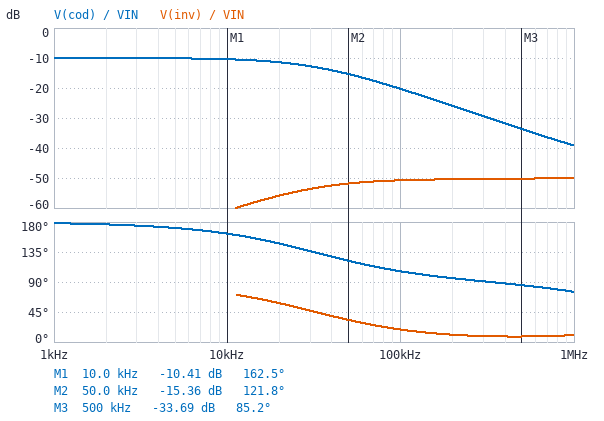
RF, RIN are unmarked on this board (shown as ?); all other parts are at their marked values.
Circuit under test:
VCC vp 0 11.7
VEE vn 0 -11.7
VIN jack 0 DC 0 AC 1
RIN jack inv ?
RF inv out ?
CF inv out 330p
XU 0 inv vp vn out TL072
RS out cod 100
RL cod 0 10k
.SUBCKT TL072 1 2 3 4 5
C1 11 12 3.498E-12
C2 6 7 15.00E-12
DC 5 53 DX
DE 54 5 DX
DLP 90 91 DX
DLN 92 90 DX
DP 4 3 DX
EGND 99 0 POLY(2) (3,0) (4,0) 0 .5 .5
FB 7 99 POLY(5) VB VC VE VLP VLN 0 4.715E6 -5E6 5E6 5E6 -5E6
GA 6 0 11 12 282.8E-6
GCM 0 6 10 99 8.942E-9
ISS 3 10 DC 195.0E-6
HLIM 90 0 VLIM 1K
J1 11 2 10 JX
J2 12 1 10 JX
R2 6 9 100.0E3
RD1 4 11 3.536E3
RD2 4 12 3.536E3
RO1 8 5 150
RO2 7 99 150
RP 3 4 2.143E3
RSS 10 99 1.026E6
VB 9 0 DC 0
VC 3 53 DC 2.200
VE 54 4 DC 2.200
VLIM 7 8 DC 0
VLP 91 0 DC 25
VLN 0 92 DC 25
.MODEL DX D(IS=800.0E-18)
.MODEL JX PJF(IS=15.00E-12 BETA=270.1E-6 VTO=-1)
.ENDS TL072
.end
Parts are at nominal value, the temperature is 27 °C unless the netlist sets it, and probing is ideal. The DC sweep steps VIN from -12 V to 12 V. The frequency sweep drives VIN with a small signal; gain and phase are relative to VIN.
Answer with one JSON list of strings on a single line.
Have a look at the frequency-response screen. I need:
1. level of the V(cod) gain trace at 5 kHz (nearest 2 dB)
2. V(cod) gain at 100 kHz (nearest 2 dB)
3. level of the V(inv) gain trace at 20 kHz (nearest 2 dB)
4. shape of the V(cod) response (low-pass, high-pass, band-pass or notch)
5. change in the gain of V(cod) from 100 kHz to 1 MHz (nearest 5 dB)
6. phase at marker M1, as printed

["-10 dB", "-20 dB", "-56 dB", "low-pass", "-20 dB", "162.5 deg"]
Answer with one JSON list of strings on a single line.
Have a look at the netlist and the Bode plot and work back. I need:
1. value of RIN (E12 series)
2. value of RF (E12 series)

["47 kΩ", "15 kΩ"]
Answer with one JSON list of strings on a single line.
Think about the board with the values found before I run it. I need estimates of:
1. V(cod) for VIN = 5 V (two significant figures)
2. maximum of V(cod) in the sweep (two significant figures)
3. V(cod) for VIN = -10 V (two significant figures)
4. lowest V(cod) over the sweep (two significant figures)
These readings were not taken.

["-1.6 V", "3.8 V", "3.2 V", "-3.8 V"]
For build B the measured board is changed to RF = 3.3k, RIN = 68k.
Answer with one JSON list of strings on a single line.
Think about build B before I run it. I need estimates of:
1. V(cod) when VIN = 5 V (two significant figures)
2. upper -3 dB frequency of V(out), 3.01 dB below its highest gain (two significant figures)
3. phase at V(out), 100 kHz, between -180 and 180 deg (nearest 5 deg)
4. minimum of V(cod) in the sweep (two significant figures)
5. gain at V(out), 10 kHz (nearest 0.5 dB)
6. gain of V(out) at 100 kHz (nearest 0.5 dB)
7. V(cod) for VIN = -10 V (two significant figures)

["-240 mV", "150 kHz", "145 deg", "-580 mV", "-26.5 dB", "-28.0 dB", "480 mV"]
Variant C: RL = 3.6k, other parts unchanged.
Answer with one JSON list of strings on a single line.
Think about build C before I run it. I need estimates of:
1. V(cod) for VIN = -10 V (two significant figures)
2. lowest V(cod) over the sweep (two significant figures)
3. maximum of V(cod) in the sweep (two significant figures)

["3.1 V", "-3.7 V", "3.7 V"]
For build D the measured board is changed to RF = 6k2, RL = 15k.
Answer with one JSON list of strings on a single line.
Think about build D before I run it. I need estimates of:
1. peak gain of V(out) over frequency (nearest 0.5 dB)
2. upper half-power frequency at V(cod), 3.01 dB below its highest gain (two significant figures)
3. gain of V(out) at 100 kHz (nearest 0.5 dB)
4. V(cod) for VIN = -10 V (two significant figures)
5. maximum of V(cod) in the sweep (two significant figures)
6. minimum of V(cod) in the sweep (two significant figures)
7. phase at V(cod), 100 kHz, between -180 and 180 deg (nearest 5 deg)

["-17.5 dB", "78 kHz", "-22.0 dB", "1.3 V", "1.6 V", "-1.6 V", "125 deg"]
